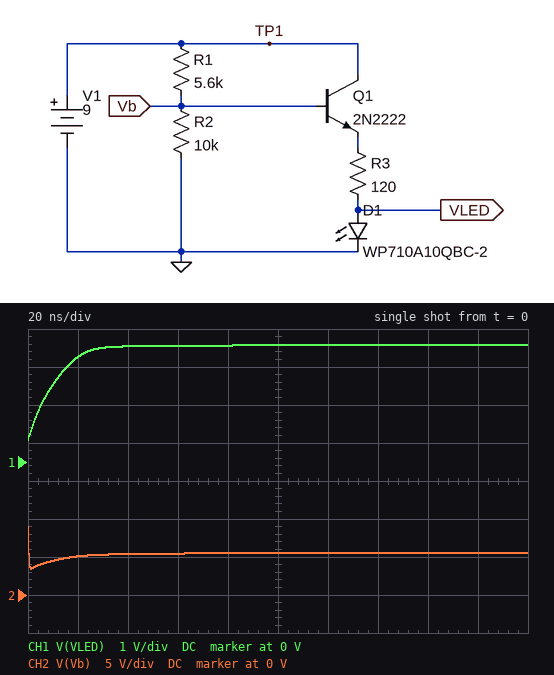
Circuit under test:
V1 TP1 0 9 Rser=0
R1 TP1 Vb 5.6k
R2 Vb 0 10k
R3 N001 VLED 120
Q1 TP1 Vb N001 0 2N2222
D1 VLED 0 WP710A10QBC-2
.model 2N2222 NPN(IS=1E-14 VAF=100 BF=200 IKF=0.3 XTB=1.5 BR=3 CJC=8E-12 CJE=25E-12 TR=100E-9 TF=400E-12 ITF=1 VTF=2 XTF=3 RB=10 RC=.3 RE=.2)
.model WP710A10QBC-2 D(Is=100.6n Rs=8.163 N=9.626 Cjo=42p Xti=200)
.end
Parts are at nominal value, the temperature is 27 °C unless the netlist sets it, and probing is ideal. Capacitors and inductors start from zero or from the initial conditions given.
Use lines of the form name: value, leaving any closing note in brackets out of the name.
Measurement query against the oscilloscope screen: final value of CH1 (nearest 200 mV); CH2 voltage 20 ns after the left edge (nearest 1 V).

final value of CH1: 3.0 V
CH2 voltage 20 ns after the left edge: 5 V
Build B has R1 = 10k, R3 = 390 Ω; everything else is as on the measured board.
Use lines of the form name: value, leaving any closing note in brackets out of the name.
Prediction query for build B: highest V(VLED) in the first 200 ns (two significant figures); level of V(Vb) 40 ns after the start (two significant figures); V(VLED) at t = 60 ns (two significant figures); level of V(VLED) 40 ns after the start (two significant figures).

highest V(VLED) in the first 200 ns: 2.6 V
level of V(Vb) 40 ns after the start: 4.5 V
V(VLED) at t = 60 ns: 2.5 V
level of V(VLED) 40 ns after the start: 2.3 V
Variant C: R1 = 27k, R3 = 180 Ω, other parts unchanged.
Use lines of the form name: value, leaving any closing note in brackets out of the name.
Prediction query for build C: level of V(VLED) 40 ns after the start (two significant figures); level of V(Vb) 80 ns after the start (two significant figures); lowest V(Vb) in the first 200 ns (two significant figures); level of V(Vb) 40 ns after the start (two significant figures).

level of V(VLED) 40 ns after the start: 2.3 V
level of V(Vb) 80 ns after the start: 2.9 V
lowest V(Vb) in the first 200 ns: 2.5 V
level of V(Vb) 40 ns after the start: 3.3 V
